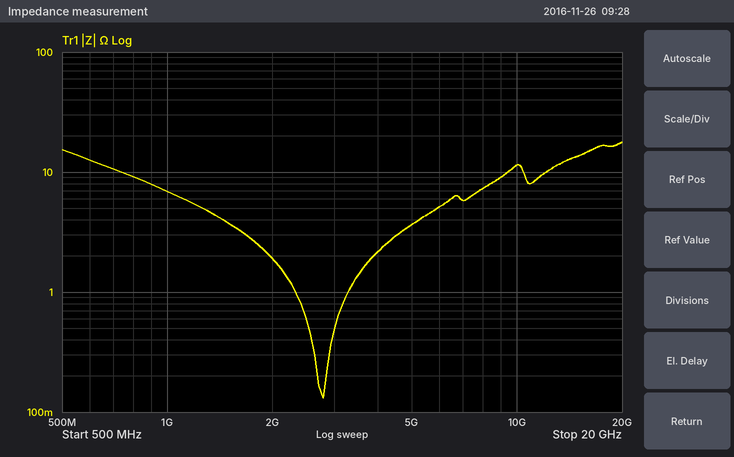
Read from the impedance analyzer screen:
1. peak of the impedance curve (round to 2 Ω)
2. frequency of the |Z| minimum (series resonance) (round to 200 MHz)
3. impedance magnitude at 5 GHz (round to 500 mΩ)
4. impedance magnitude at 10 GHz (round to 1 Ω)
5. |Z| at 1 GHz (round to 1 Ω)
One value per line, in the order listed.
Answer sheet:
18 Ω
2.8 GHz
3.5 Ω
11 Ω
7 Ω
